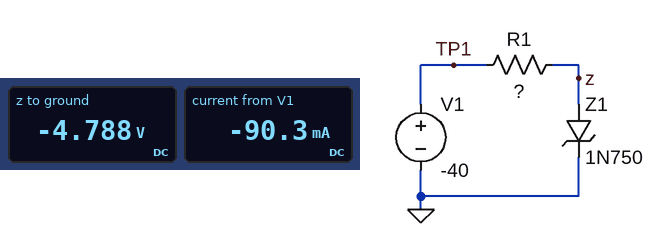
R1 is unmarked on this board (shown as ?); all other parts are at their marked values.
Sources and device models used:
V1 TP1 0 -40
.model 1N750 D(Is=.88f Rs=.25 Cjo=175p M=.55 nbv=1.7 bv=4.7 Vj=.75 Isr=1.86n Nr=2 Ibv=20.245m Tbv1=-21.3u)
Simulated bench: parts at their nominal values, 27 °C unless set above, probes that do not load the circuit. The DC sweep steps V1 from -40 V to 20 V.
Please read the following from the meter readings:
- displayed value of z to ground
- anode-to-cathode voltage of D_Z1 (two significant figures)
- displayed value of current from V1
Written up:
-4.788 V
-4.8 V
-90.3 mA
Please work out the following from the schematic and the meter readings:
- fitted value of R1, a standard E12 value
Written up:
390 Ω
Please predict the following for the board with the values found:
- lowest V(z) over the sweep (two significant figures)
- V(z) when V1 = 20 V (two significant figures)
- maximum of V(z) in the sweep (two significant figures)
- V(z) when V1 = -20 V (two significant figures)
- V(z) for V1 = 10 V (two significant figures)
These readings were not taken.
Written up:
-4.8 V
830 mV
830 mV
-4.7 V
800 mV
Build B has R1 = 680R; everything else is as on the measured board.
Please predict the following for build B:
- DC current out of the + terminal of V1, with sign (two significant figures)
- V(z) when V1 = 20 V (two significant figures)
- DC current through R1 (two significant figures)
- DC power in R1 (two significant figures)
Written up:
-52 mA
810 mV
52 mA
1.8 W
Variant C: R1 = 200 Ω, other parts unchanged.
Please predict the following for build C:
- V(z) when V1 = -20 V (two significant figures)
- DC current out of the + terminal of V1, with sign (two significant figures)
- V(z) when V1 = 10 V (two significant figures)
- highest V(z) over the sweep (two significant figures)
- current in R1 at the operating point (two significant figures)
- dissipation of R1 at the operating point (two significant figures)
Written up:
-4.8 V
-180 mA
830 mV
860 mV
180 mA
6.2 W
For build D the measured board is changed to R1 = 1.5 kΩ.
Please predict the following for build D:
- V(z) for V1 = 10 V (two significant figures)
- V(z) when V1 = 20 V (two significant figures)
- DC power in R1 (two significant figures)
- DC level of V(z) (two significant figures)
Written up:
760 mV
780 mV
830 mW
-4.7 V
